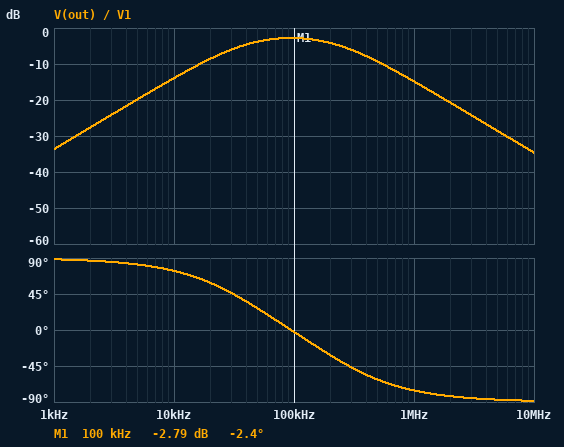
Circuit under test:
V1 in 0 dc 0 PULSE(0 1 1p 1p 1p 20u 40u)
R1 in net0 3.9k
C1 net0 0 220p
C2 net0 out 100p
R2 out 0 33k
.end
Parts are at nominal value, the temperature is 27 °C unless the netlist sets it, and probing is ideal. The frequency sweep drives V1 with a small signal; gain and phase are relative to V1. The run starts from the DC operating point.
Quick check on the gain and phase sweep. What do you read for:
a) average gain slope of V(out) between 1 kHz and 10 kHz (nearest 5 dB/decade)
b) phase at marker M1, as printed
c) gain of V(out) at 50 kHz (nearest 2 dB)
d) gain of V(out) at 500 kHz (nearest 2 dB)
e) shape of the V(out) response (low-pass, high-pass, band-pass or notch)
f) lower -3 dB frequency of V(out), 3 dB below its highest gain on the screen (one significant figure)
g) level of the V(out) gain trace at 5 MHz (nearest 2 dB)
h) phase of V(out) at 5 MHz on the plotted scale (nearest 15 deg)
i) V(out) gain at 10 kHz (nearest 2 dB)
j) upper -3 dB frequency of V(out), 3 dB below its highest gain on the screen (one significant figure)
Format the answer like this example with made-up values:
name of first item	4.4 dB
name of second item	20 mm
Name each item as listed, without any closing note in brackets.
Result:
average gain slope of V(out) between 1 kHz and 10 kHz	20 dB/decade
phase at marker M1, as printed	-2.4 deg
gain of V(out) at 50 kHz	-4 dB
gain of V(out) at 500 kHz	-10 dB
shape of the V(out) response	band-pass
lower -3 dB frequency of V(out), 3 dB below its highest gain on the screen	30 kHz
level of the V(out) gain trace at 5 MHz	-28 dB
phase of V(out) at 5 MHz on the plotted scale	-90 deg
V(out) gain at 10 kHz	-14 dB
upper -3 dB frequency of V(out), 3 dB below its highest gain on the screen	300 kHz
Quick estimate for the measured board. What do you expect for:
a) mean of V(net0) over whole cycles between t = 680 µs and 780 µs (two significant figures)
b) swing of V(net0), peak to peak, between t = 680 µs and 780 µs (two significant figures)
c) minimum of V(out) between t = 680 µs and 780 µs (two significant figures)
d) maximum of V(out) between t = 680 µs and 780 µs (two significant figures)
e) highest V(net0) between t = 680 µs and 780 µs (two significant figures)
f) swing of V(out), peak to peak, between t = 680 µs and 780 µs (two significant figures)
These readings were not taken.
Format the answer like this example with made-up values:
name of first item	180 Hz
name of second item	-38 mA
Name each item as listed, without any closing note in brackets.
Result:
mean of V(net0) over whole cycles between t = 680 µs and 780 µs	500 mV
swing of V(net0), peak to peak, between t = 680 µs and 780 µs	1.0 V
minimum of V(out) between t = 680 µs and 780 µs	-580 mV
maximum of V(out) between t = 680 µs and 780 µs	580 mV
highest V(net0) between t = 680 µs and 780 µs	1.0 V
swing of V(out), peak to peak, between t = 680 µs and 780 µs	1.2 V
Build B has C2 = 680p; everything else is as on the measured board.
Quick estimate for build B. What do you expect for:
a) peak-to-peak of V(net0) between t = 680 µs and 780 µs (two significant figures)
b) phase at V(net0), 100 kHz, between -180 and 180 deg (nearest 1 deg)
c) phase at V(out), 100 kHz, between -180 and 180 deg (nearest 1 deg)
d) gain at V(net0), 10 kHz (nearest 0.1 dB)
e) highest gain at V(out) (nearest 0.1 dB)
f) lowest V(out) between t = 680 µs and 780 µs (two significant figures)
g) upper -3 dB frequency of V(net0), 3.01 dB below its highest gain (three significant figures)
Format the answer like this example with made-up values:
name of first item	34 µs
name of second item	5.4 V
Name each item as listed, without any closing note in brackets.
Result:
peak-to-peak of V(net0) between t = 680 µs and 780 µs	930 mV
phase at V(net0), 100 kHz, between -180 and 180 deg	-26 deg
phase at V(out), 100 kHz, between -180 and 180 deg	-22 deg
gain at V(net0), 10 kHz	-0.7 dB
highest gain at V(out)	-1.3 dB
lowest V(out) between t = 680 µs and 780 µs	-540 mV
upper -3 dB frequency of V(net0), 3.01 dB below its highest gain	160 kHz
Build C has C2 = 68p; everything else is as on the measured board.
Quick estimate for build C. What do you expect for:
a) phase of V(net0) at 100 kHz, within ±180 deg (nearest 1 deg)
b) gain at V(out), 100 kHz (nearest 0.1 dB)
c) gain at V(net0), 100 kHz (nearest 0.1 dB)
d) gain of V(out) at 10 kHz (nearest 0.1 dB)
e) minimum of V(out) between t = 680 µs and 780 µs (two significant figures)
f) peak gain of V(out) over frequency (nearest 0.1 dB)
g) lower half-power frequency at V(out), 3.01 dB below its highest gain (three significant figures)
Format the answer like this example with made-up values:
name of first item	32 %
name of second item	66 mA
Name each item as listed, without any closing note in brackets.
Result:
phase of V(net0) at 100 kHz, within ±180 deg	-29 deg
gain at V(out), 100 kHz	-3.6 dB
gain at V(net0), 100 kHz	-1.8 dB
gain of V(out) at 10 kHz	-17.1 dB
minimum of V(out) between t = 680 µs and 780 µs	-520 mV
peak gain of V(out) over frequency	-3.5 dB
lower half-power frequency at V(out), 3.01 dB below its highest gain	41.2 kHz
